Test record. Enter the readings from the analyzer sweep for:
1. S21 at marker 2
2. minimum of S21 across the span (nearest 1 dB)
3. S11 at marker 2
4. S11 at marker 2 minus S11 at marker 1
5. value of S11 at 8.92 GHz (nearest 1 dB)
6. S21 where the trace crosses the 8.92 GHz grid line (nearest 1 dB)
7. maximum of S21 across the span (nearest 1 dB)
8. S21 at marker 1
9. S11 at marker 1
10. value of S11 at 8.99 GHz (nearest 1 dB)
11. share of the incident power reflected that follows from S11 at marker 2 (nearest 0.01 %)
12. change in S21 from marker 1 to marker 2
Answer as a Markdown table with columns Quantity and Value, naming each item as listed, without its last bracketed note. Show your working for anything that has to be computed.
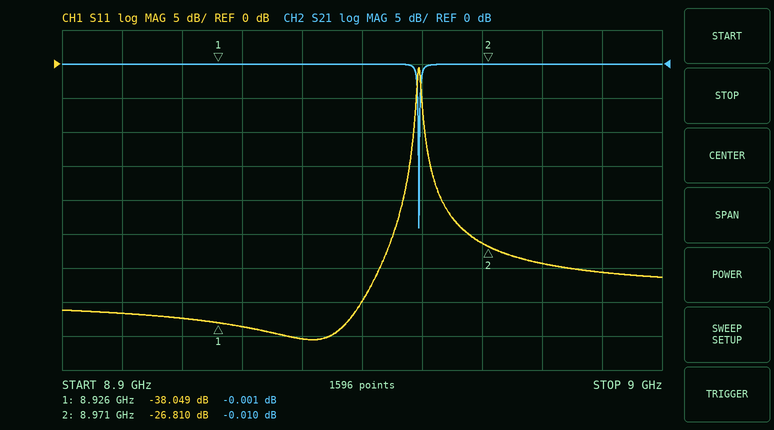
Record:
| Quantity | Value |
|---|---|
| S21 at marker 2 | -0.010 dB |
| minimum of S21 across the span | -24 dB |
| S11 at marker 2 | -26.810 dB |
| S11 at marker 2 minus S11 at marker 1 | -26.81 − (-38.049) = 11.239 dB |
| value of S11 at 8.92 GHz | -37 dB |
| S21 where the trace crosses the 8.92 GHz grid line | 0 dB |
| maximum of S21 across the span | 0 dB |
| S21 at marker 1 | -0.001 dB |
| S11 at marker 1 | -38.049 dB |
| value of S11 at 8.99 GHz | -31 dB |
| share of the incident power reflected that follows from S11 at marker 2 | 10^(-26.81/10) ≈ 0.21 % |
| change in S21 from marker 1 to marker 2 | -0.01 − (-0.001) = -0.009 dB |
